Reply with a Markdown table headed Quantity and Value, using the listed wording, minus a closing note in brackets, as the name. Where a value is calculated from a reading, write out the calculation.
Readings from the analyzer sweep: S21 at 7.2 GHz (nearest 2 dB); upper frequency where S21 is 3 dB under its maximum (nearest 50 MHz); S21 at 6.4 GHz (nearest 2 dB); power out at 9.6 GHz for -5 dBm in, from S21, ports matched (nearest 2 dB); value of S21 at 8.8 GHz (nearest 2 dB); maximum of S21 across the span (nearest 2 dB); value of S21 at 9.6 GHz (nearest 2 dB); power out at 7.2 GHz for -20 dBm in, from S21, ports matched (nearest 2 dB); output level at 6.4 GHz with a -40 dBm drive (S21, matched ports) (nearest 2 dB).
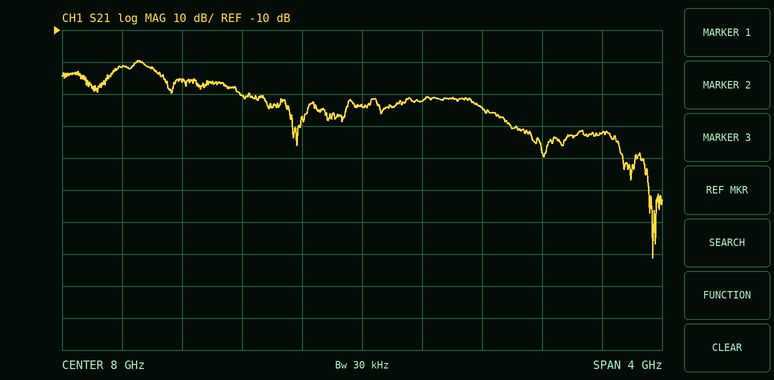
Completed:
| Quantity | Value |
|---|---|
| S21 at 7.2 GHz | -30 dB |
| upper frequency where S21 is 3 dB under its maximum | 6.60 GHz |
| S21 at 6.4 GHz | -22 dB |
| power out at 9.6 GHz for -5 dBm in, from S21, ports matched | -5 dBm + (-42 dB) = -48 dBm |
| value of S21 at 8.8 GHz | -34 dB |
| maximum of S21 across the span | -20 dB |
| value of S21 at 9.6 GHz | -42 dB |
| power out at 7.2 GHz for -20 dBm in, from S21, ports matched | -20 dBm + (-30 dB) = -50 dBm |
| output level at 6.4 GHz with a -40 dBm drive (S21, matched ports) | -40 dBm + (-22 dB) = -62 dBm |
